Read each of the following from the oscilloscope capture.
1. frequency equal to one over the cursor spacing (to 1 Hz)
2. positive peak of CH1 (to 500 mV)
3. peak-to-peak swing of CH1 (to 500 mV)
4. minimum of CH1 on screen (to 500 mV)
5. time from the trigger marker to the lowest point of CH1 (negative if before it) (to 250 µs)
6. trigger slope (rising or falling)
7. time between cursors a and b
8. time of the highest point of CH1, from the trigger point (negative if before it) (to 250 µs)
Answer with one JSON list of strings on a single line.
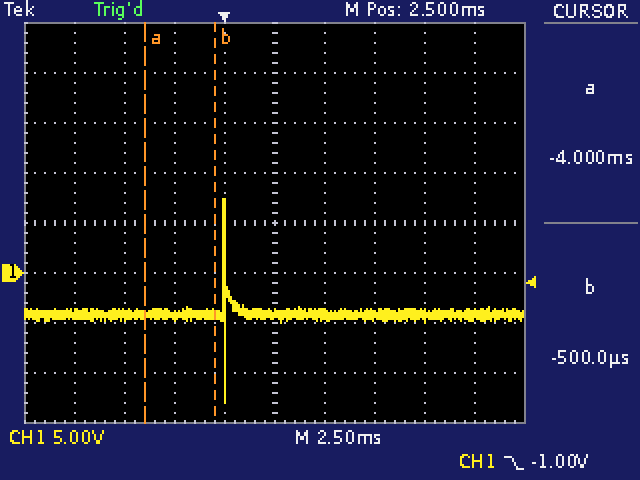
["286 Hz", "7.5 V", "20.5 V", "-13.0 V", "0.00 ms", "falling", "3.50 ms", "0.00 ms"]
